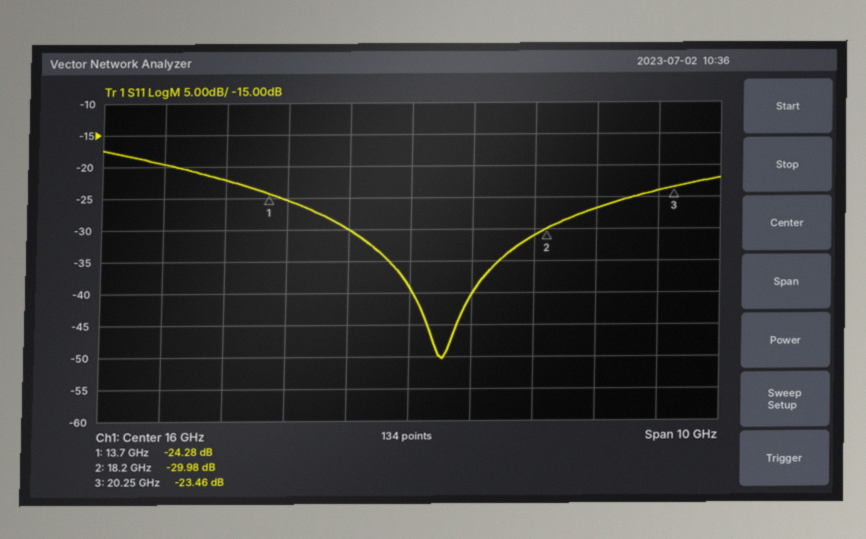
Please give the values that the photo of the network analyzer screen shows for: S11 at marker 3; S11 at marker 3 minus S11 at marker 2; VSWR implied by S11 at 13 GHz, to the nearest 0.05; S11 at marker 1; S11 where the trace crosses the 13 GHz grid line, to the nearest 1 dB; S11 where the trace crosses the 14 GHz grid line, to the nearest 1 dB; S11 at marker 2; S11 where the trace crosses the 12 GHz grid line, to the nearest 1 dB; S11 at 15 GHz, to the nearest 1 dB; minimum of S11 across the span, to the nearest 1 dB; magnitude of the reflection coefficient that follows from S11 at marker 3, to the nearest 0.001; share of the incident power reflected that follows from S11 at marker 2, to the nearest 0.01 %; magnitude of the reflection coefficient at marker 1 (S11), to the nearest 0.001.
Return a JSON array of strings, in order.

["-23.46 dB", "6.52 dB", "1.15", "-24.28 dB", "-22 dB", "-25 dB", "-29.98 dB", "-20 dB", "-30 dB", "-50 dB", "0.067", "0.10 %", "0.061"]
